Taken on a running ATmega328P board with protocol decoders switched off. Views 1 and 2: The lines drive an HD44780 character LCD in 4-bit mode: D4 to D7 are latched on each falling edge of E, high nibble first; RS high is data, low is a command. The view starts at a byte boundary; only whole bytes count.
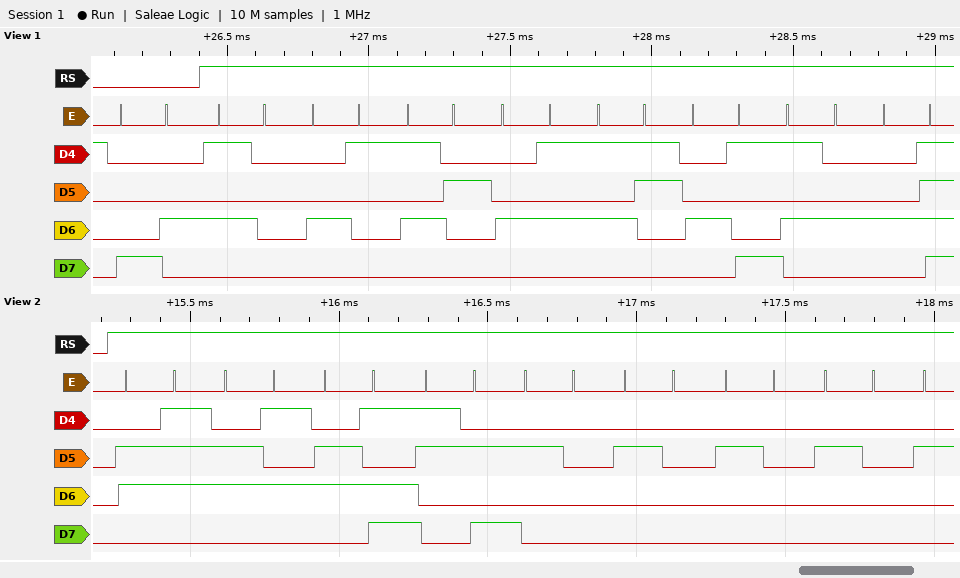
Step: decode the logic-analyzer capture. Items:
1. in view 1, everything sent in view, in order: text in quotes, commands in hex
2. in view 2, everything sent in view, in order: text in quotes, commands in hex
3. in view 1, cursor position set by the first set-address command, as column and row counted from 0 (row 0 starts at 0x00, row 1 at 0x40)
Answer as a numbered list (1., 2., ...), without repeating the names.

1. 0x84 "PARESITO"
2. "gem:    "
3. column 4, row 0
